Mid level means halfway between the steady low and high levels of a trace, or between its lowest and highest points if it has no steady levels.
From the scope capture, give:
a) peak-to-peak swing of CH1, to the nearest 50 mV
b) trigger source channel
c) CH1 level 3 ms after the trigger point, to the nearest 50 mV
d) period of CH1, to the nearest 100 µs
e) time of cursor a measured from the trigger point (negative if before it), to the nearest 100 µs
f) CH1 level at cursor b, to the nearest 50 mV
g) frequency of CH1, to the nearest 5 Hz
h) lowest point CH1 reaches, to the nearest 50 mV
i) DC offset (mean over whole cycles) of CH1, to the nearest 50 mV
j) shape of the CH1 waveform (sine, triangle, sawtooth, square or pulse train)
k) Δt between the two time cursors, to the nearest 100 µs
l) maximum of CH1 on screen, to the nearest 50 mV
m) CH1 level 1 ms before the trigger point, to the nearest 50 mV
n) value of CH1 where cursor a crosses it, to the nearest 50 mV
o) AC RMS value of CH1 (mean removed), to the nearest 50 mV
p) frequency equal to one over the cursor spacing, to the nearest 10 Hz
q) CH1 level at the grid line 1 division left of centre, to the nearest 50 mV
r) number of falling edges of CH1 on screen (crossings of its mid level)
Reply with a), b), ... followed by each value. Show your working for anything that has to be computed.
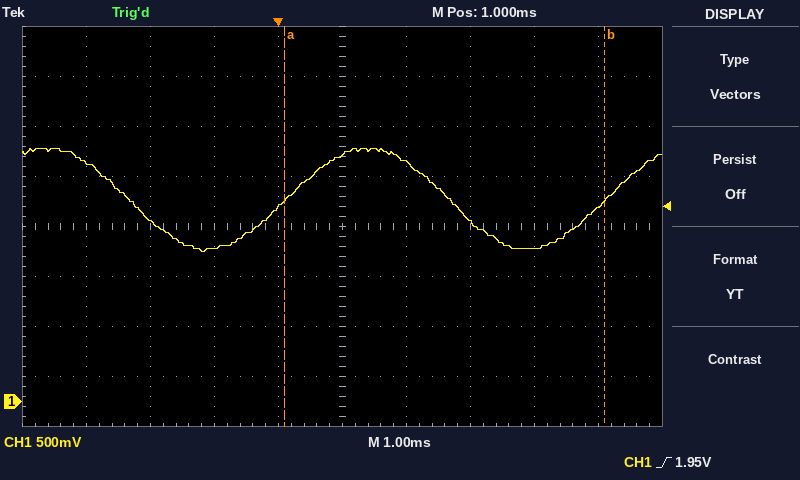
a) 2.55 V − (1.50 V) = 1.05 V
b) CH1
c) 1.80 V
d) 5.0 ms
e) +100 µs
f) 2.00 V
g) 1 / 5.0 ms ≈ 200 Hz
h) 1.50 V
i) (2.55 V + (1.50 V)) / 2 ≈ 2.03 V, so 2.05 V to the nearest 50 mV
j) sine
k) 5.0 ms
l) 2.55 V
m) 1.55 V
n) 2.00 V
o) 1.05 V / (2√2) ≈ 371 mV, so 350 mV to the nearest 50 mV
p) 1 / 5.0 ms ≈ 200 Hz
q) 1.95 V
r) 2
